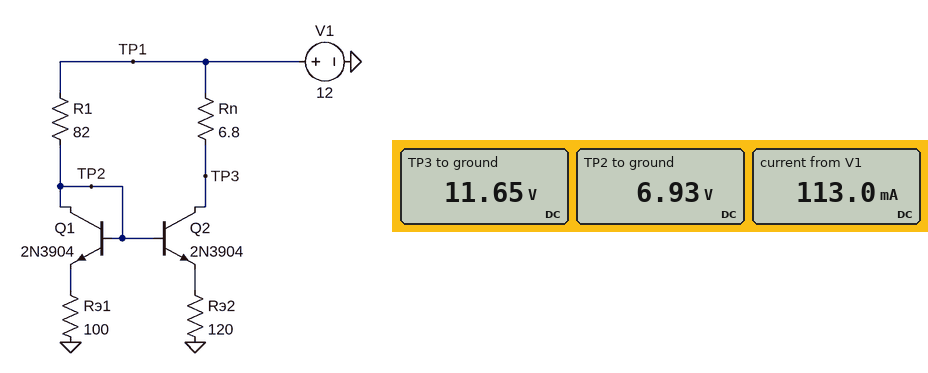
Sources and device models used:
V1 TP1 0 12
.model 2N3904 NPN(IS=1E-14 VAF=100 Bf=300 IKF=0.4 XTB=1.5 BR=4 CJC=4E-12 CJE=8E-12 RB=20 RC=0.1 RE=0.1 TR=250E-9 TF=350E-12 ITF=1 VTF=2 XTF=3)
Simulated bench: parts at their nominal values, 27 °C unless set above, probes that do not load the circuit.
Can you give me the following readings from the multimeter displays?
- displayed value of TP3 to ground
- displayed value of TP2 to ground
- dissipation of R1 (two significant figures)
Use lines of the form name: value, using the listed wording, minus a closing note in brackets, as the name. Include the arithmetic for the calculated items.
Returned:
displayed value of TP3 to ground: 11.65 V
displayed value of TP2 to ground: 6.93 V
dissipation of R1: (12 V - 6.93 V)^2 / 82 Ω = 310 mW
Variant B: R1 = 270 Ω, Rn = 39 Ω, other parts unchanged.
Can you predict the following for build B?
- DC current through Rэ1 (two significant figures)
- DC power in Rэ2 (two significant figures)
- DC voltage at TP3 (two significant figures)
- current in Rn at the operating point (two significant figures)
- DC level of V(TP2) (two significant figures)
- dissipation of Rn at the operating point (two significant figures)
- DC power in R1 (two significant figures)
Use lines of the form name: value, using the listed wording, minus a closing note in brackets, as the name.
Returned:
DC current through Rэ1: 30 mA
DC power in Rэ2: 77 mW
DC voltage at TP3: 11 V
current in Rn at the operating point: 25 mA
DC level of V(TP2): 3.8 V
dissipation of Rn at the operating point: 25 mW
DC power in R1: 250 mW
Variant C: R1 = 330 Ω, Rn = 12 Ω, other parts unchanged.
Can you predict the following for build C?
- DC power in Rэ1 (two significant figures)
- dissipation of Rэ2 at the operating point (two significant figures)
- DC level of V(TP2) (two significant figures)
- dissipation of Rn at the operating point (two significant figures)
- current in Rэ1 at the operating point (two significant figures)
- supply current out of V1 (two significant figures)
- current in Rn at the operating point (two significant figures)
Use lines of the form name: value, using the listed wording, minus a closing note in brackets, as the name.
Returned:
DC power in Rэ1: 68 mW
dissipation of Rэ2 at the operating point: 57 mW
DC level of V(TP2): 3.4 V
dissipation of Rn at the operating point: 5.7 mW
current in Rэ1 at the operating point: 26 mA
supply current out of V1: 48 mA
current in Rn at the operating point: 22 mA
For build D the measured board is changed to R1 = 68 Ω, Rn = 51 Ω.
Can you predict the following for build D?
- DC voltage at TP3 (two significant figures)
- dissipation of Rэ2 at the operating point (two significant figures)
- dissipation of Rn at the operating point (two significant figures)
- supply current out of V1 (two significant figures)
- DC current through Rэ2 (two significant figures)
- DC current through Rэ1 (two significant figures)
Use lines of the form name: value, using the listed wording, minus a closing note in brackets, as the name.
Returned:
DC voltage at TP3: 9.2 V
dissipation of Rэ2 at the operating point: 370 mW
dissipation of Rn at the operating point: 160 mW
supply current out of V1: 120 mA
DC current through Rэ2: 56 mA
DC current through Rэ1: 67 mA
